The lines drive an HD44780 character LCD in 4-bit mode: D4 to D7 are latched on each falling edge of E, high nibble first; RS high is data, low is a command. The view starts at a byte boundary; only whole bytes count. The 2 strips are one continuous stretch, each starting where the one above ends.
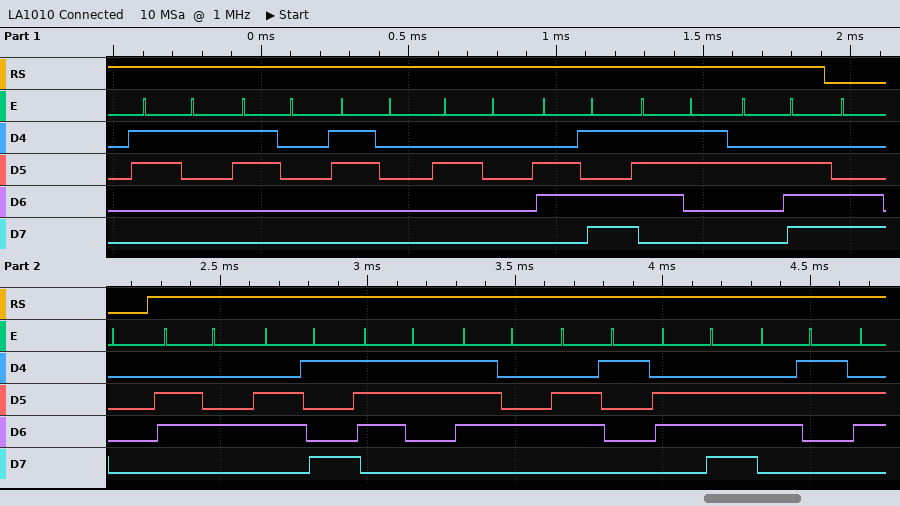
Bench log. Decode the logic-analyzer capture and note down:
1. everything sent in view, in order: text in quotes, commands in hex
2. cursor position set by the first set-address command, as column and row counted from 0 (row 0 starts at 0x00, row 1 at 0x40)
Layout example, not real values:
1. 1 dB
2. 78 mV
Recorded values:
1. "100 ms." 0xC0 "distanc"
2. column 0, row 1
